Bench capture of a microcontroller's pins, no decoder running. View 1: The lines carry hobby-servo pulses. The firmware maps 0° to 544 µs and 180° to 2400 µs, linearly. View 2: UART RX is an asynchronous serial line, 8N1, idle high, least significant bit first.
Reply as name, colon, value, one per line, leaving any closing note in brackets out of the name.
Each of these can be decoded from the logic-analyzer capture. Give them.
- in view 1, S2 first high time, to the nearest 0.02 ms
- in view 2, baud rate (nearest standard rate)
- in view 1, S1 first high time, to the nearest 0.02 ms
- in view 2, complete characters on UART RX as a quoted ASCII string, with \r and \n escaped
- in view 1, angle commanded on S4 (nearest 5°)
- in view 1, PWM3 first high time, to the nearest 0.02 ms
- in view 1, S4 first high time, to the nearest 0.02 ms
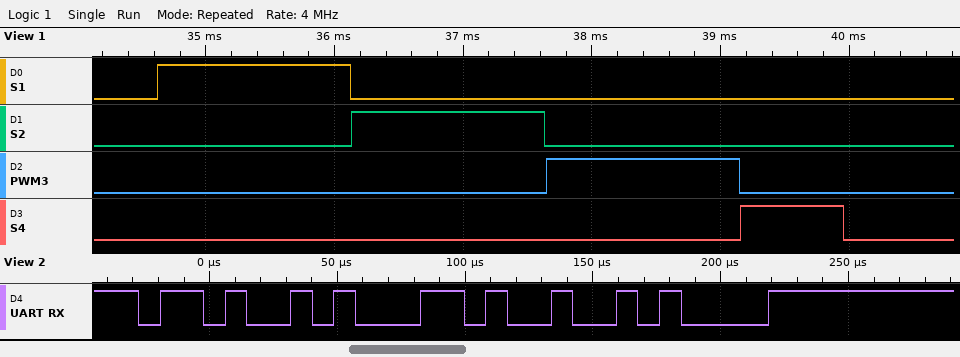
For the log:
in view 1, S2 first high time, to the nearest 0.02 ms: 1.50 ms
in view 2, baud rate: 115200 baud
in view 1, S1 first high time, to the nearest 0.02 ms: 1.50 ms
in view 2, complete characters on UART RX as a quoted ASCII string, with \r and \n escaped: "K,\n"
in view 1, angle commanded on S4: 25°
in view 1, PWM3 first high time, to the nearest 0.02 ms: 1.50 ms
in view 1, S4 first high time, to the nearest 0.02 ms: 0.80 ms
